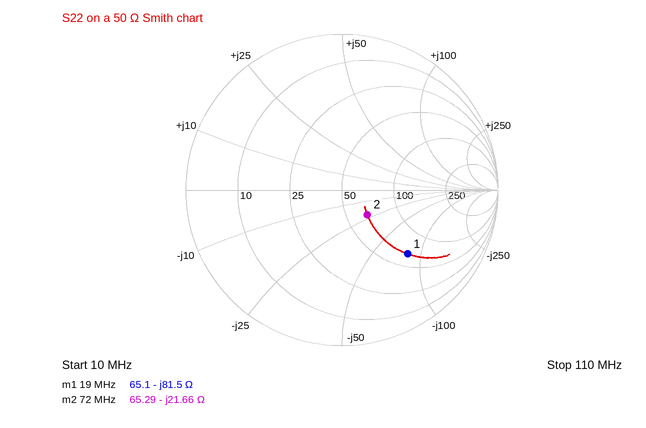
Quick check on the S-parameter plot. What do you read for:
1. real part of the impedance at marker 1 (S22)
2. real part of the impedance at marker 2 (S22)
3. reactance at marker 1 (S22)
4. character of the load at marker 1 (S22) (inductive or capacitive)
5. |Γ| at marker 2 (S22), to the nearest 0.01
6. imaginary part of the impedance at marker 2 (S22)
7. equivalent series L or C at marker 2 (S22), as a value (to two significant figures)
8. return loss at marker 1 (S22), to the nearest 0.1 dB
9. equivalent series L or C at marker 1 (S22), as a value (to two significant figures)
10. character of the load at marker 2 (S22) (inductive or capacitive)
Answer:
65.1 Ω
65.29 Ω
-81.5 Ω
capacitive
0.23
-21.66 Ω
100 pF
4.6 dB
100 pF
capacitive
